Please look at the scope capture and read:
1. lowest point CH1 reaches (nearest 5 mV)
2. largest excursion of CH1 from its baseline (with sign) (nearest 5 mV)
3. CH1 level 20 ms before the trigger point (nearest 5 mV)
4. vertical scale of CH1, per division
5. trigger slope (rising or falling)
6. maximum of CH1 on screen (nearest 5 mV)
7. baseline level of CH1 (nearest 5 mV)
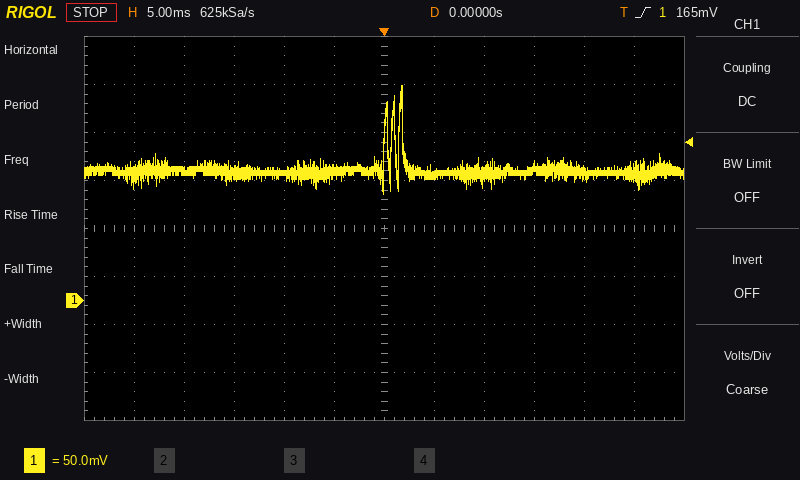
110 mV
+90 mV
135 mV
50 mV
rising
225 mV
135 mV
